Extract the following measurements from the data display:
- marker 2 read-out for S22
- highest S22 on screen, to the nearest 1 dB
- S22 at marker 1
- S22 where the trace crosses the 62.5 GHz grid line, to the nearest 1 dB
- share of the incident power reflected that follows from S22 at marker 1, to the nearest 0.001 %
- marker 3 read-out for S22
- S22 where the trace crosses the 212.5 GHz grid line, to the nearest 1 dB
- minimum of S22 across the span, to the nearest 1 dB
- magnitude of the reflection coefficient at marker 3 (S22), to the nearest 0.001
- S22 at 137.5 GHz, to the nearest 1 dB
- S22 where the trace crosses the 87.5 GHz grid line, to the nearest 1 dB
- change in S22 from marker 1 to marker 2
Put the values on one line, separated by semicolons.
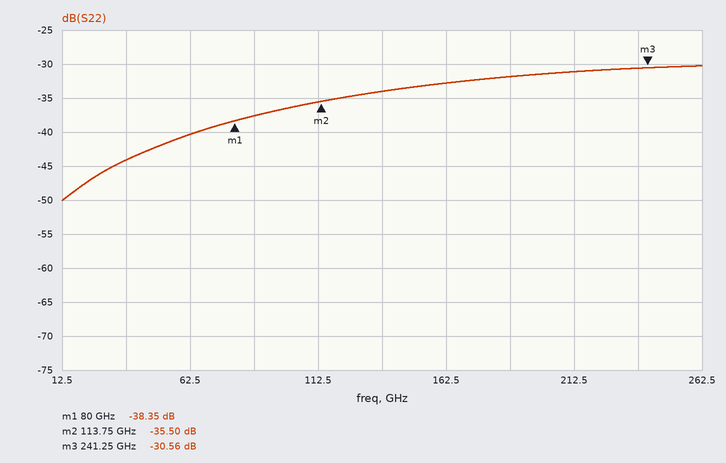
-35.50 dB; -30 dB; -38.35 dB; -40 dB; 0.015 %; -30.56 dB; -31 dB; -50 dB; 0.030; -34 dB; -38 dB; 2.85 dB
